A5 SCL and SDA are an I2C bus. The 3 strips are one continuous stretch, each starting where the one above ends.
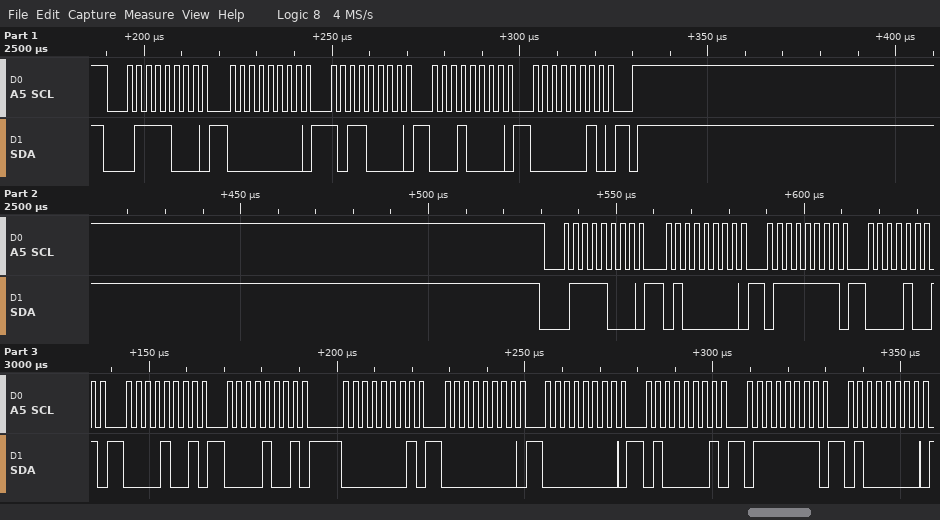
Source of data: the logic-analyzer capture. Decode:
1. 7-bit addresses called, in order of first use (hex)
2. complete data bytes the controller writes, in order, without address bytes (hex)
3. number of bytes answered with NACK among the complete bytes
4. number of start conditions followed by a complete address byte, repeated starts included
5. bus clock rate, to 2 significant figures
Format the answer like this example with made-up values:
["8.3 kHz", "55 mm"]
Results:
["0x3C", "00 B0 10 02 40 7F 09 09 09 01 00 00 41 7F 40", "0", "2", "400 kHz"]
